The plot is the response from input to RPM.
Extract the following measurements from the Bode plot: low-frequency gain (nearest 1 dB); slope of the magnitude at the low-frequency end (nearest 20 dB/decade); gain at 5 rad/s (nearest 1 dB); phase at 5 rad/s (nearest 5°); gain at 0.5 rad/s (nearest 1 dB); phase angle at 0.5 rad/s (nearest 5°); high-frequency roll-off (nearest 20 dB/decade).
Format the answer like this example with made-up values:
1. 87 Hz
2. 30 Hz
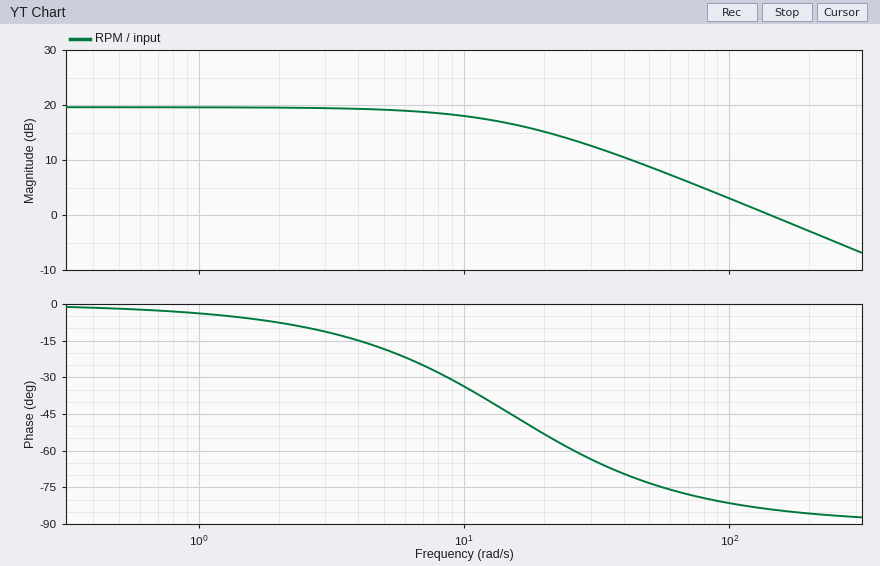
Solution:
1. 20 dB
2. 0 dB/decade
3. 19 dB
4. -20°
5. 20 dB
6. 0°
7. -20 dB/decade
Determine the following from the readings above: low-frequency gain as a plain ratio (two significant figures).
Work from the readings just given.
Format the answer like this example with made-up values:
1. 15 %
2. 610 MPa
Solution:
1. 10
